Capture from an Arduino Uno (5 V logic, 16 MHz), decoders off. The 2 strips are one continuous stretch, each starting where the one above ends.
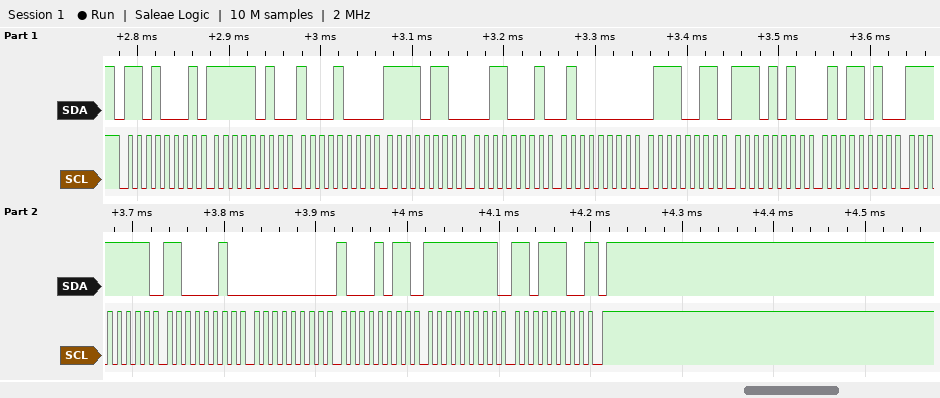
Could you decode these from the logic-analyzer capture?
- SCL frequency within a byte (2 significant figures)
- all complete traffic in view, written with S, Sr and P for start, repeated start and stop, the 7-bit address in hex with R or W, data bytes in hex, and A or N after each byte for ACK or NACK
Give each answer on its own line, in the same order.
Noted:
100 kHz
S 68R A FA A 88 A F6 A 31 A 40 A 73 A EA A 5A A FF A C2 A 00 A 8B A FF A DC N P
